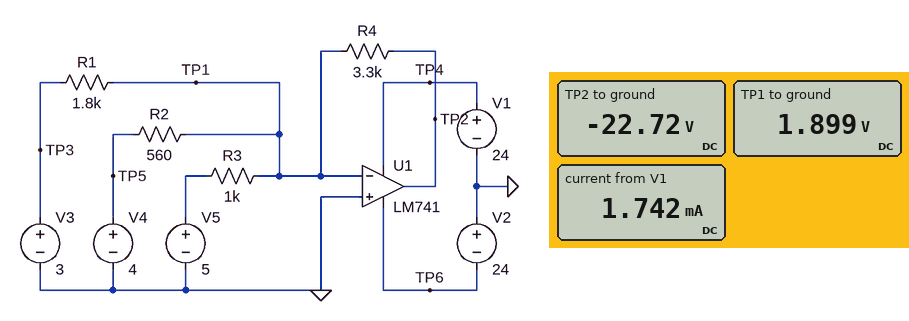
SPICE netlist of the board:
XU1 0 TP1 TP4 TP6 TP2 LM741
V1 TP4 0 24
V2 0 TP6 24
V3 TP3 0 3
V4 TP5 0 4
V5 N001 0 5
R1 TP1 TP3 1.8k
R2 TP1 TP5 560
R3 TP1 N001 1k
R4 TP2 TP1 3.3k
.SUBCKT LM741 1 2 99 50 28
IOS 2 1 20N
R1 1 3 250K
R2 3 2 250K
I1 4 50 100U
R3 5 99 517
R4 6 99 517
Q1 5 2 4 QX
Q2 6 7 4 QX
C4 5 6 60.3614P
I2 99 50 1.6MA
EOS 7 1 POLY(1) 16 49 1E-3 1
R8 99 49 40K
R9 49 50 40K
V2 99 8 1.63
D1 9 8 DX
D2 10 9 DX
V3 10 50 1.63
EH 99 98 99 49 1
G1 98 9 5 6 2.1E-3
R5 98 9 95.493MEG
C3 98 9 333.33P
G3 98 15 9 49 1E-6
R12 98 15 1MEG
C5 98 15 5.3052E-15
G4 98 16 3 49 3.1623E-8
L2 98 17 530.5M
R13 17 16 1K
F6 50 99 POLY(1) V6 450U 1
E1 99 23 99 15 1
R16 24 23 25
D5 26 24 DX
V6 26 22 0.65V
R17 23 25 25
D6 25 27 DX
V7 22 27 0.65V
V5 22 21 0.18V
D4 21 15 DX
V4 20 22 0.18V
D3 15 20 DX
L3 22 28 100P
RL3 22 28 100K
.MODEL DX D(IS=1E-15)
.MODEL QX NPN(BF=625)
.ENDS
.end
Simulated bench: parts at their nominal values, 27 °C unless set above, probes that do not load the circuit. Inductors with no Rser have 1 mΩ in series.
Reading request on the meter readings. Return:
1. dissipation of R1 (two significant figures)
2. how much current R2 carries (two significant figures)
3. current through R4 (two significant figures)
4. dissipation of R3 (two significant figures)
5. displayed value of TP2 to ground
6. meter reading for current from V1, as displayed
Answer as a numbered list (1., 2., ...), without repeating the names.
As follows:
1. 670 µW
2. 3.8 mA
3. 7.5 mA
4. 9.6 mW
5. -22.72 V
6. 1.742 mA
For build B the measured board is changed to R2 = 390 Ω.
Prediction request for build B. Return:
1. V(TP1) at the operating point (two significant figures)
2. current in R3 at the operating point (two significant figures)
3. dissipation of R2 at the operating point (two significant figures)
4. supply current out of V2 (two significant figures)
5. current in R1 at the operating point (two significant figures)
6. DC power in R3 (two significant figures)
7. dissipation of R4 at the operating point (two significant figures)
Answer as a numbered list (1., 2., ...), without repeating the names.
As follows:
1. 2.3 V
2. 2.7 mA
3. 7.7 mW
4. 9.3 mA
5. 410 µA
6. 7.5 mW
7. 190 mW
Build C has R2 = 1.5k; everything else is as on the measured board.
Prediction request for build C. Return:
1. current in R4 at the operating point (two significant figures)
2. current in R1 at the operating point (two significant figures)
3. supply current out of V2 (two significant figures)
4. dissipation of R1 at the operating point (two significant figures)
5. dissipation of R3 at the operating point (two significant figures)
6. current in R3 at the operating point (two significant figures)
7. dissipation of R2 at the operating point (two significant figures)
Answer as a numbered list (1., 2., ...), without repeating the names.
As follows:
1. 7.2 mA
2. 1.1 mA
3. 8.9 mA
4. 2.3 mW
5. 16 mW
6. 4.0 mA
7. 6.1 mW
